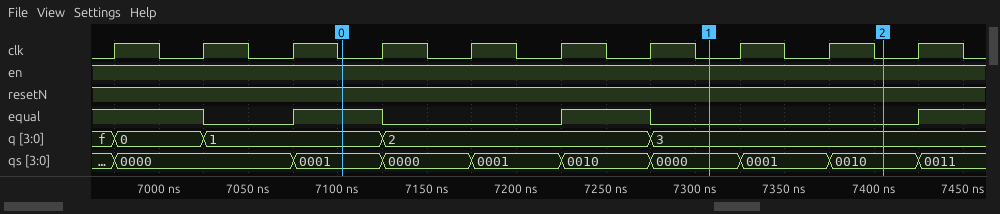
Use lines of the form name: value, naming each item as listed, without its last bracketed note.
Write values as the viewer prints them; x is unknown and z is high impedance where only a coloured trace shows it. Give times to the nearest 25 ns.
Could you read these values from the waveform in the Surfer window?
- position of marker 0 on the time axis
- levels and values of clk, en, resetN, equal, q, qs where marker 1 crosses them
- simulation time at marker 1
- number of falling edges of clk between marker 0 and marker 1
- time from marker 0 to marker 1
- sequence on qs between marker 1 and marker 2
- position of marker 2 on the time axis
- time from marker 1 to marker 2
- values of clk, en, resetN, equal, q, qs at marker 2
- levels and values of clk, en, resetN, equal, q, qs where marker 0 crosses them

position of marker 0 on the time axis: 7100 ns
levels and values of clk, en, resetN, equal, q, qs where marker 1 crosses them: clk=0, en=1, resetN=1, equal=0, q=3, qs=0000
simulation time at marker 1: 7300 ns
number of falling edges of clk between marker 0 and marker 1: 4
time from marker 0 to marker 1: 200 ns
sequence on qs between marker 1 and marker 2: 0000, 0001, 0010
position of marker 2 on the time axis: 7400 ns
time from marker 1 to marker 2: 100 ns
values of clk, en, resetN, equal, q, qs at marker 2: clk=0, en=1, resetN=1, equal=0, q=3, qs=0010
levels and values of clk, en, resetN, equal, q, qs where marker 0 crosses them: clk=0, en=1, resetN=1, equal=1, q=1, qs=0001
